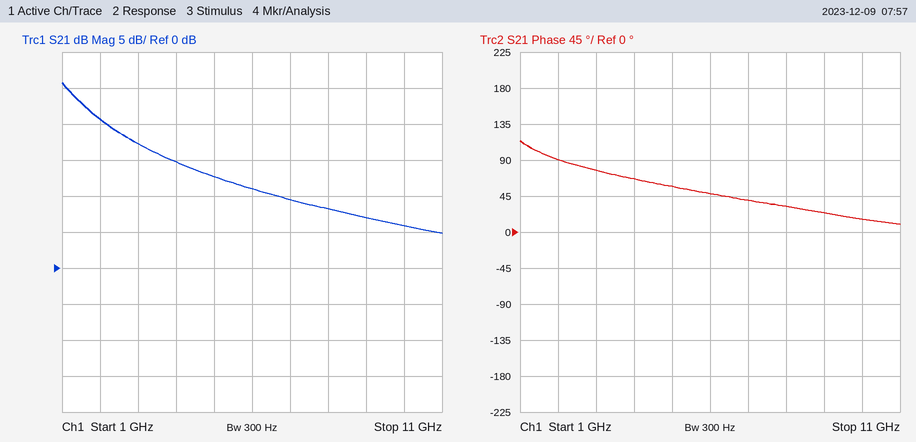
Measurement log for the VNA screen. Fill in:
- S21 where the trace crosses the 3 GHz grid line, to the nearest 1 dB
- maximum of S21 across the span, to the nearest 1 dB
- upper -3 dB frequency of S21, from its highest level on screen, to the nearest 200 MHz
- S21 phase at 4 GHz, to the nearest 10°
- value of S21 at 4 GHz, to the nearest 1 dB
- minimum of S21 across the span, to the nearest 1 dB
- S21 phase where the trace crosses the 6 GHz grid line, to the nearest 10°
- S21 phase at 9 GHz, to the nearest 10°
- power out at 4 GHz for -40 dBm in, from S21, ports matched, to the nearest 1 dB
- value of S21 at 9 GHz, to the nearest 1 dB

17 dB
26 dB
1.6 GHz
70°
15 dB
5 dB
50°
20°
-25 dBm
7 dB
